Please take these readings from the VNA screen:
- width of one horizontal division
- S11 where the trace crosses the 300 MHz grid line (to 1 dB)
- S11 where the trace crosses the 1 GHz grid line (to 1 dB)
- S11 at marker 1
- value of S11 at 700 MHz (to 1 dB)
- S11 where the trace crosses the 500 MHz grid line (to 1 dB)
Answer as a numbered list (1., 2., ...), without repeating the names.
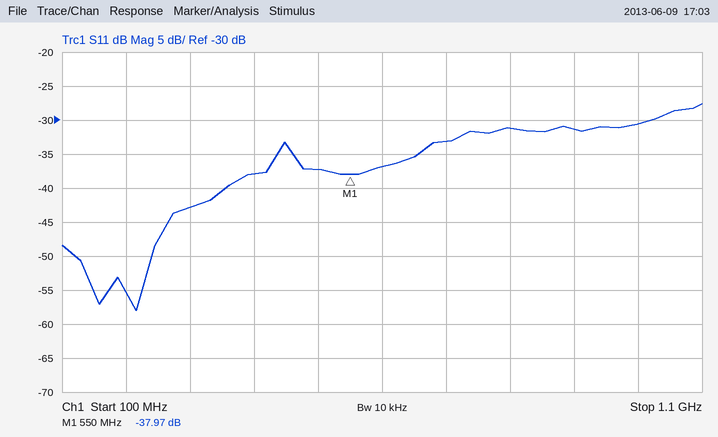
1. 100 MHz
2. -43 dB
3. -31 dB
4. -37.97 dB
5. -33 dB
6. -37 dB
